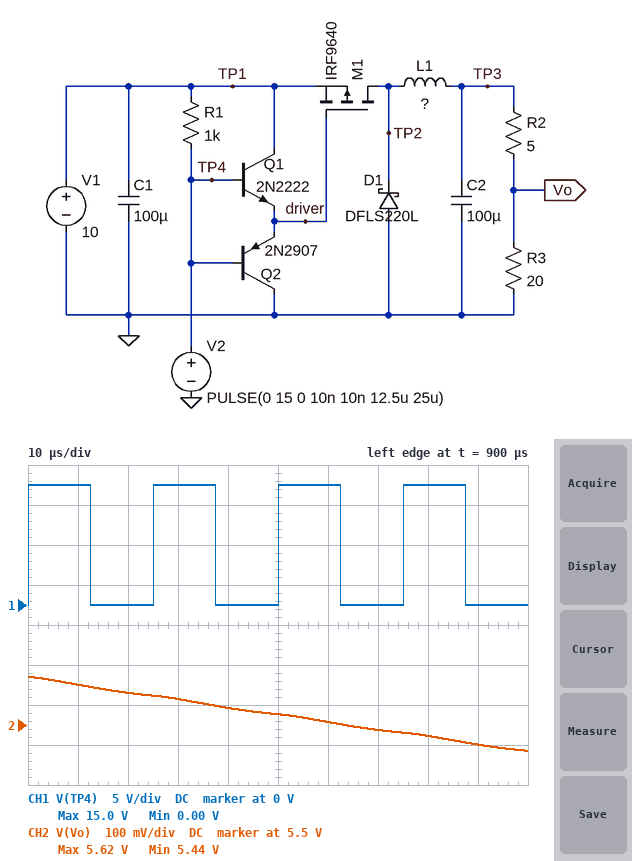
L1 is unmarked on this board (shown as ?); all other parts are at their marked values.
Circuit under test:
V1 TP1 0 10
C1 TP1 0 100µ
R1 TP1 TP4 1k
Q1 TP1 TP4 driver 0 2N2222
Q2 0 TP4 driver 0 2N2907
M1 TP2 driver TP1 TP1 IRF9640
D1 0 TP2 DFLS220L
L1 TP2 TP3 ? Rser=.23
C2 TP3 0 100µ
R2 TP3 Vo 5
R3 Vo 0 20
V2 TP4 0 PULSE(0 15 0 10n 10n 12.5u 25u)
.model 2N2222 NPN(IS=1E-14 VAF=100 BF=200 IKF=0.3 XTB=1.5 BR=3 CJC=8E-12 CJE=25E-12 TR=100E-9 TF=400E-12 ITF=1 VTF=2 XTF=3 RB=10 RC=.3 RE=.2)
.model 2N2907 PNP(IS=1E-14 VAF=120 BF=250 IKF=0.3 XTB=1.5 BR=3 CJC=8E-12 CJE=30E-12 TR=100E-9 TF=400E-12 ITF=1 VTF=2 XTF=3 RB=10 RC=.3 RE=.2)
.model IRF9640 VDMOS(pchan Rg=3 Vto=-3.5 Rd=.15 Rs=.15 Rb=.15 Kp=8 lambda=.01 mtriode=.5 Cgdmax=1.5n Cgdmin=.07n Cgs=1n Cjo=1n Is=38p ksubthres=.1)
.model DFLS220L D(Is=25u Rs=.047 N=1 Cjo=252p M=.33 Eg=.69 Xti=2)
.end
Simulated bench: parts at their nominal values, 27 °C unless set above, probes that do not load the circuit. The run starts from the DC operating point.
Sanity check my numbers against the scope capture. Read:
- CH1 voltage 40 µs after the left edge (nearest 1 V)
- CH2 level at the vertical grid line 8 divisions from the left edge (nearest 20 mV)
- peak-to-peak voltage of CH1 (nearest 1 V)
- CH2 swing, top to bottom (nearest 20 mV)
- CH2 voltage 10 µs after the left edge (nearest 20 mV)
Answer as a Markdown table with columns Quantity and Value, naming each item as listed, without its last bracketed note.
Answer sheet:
| Quantity | Value |
|---|---|
| CH1 voltage 40 µs after the left edge | 0 V |
| CH2 level at the vertical grid line 8 divisions from the left edge | 5.48 V |
| peak-to-peak voltage of CH1 | 15 V |
| CH2 swing, top to bottom | 180 mV |
| CH2 voltage 10 µs after the left edge | 5.60 V |
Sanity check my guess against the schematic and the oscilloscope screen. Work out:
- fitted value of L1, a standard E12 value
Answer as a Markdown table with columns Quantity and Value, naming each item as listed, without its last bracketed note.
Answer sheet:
| Quantity | Value |
|---|---|
| fitted value of L1, a standard E12 value | 270 µH |
